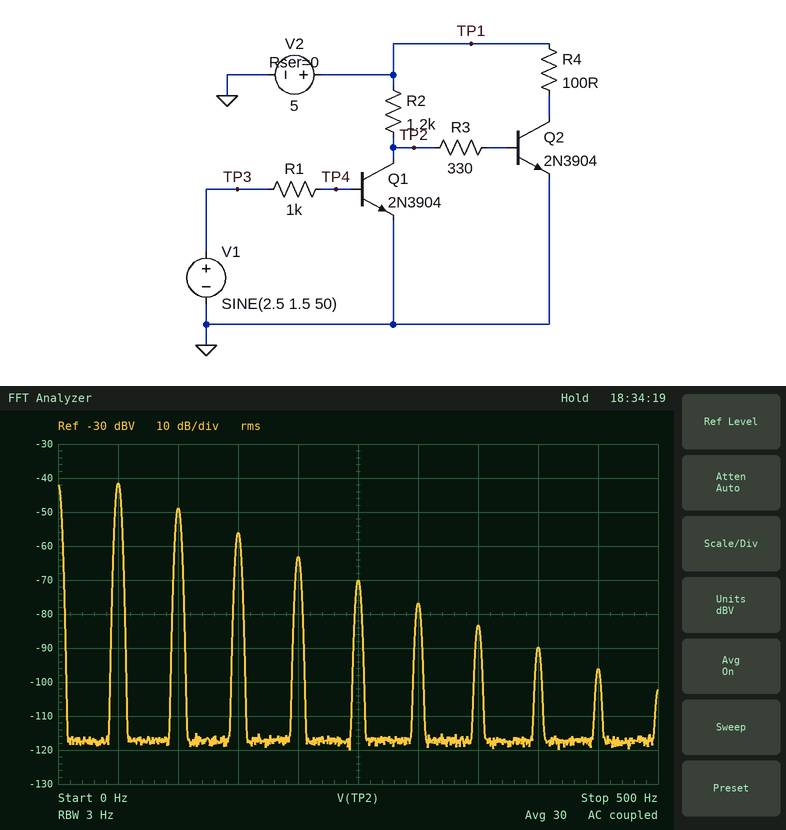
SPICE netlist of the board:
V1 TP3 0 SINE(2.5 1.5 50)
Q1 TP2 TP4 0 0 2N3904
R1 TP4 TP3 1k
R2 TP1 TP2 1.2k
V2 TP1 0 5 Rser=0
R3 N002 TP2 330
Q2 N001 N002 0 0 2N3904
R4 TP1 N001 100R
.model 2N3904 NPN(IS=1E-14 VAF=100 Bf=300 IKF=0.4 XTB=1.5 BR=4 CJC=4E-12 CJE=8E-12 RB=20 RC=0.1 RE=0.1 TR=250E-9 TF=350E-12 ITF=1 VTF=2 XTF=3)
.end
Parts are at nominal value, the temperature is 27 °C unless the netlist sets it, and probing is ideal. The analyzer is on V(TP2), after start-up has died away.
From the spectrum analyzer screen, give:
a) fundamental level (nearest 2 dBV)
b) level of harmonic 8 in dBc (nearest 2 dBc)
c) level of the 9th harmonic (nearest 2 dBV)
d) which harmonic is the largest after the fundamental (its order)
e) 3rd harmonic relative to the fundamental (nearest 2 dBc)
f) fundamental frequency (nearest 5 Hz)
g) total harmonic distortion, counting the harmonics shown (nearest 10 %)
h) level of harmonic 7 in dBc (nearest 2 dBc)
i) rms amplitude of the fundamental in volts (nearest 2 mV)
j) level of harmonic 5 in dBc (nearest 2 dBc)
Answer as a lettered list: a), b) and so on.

a) -42 dBV
b) -48 dBc
c) -96 dBV
d) 2
e) -14 dBc
f) 50 Hz
g) 50 %
h) -42 dBc
i) 8 mV
j) -28 dBc
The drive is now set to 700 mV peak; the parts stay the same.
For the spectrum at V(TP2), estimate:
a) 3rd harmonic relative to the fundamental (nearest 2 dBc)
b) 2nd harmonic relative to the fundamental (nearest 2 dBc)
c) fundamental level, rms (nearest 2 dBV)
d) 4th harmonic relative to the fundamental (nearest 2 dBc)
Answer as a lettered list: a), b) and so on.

a) -30 dBc
b) -16 dBc
c) -52 dBV
d) -46 dBc
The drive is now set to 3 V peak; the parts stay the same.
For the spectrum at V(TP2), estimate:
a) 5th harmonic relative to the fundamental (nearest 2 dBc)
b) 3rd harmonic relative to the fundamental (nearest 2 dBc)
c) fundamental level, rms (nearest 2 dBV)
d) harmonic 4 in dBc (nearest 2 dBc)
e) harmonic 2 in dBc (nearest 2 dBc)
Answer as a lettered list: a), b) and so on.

a) -12 dBc
b) -16 dBc
c) -4 dBV
d) -16 dBc
e) -4 dBc
